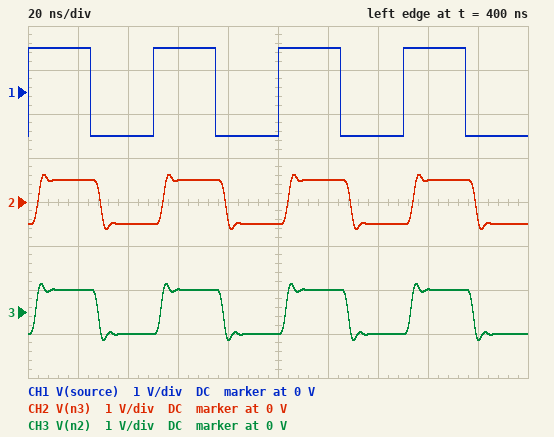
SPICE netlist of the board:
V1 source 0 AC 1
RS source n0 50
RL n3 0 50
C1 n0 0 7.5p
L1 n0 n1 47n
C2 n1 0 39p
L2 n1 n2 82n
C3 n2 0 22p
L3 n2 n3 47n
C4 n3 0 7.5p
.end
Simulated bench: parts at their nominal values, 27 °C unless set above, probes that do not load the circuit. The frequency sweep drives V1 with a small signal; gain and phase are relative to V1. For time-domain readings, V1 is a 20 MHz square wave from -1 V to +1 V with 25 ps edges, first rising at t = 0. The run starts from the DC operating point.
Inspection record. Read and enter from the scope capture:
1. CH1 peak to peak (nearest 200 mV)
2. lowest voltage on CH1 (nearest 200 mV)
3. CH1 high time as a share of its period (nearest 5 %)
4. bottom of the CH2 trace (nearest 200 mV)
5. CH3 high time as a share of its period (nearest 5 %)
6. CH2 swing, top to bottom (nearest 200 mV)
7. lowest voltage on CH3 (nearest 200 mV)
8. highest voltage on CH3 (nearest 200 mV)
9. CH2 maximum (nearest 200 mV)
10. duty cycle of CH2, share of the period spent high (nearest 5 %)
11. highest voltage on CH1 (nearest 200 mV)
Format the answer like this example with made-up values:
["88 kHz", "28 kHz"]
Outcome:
["2.0 V", "-1.0 V", "50 %", "-600 mV", "50 %", "1.2 V", "-600 mV", "600 mV", "600 mV", "50 %", "1.0 V"]
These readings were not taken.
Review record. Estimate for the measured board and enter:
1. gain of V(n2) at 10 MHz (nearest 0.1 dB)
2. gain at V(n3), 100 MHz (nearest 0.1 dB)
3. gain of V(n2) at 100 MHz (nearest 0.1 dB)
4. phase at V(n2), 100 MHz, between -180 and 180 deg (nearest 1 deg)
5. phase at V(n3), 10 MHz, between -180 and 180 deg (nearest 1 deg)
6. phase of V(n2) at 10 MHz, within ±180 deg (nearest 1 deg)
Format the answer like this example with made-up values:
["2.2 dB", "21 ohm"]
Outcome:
["-6.0 dB", "-6.3 dB", "-6.0 dB", "-103 deg", "-13 deg", "-10 deg"]
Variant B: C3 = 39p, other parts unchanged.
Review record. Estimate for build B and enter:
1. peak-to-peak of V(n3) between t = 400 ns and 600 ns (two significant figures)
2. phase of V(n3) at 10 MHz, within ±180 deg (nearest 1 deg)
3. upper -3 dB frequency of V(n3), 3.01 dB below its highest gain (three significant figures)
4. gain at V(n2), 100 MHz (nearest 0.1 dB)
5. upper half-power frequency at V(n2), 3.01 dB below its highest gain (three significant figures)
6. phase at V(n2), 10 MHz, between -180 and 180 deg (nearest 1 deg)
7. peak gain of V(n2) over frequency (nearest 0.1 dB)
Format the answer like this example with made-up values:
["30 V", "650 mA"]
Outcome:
["1.3 V", "-15 deg", "161 MHz", "-5.7 dB", "166 MHz", "-11 deg", "-5.5 dB"]
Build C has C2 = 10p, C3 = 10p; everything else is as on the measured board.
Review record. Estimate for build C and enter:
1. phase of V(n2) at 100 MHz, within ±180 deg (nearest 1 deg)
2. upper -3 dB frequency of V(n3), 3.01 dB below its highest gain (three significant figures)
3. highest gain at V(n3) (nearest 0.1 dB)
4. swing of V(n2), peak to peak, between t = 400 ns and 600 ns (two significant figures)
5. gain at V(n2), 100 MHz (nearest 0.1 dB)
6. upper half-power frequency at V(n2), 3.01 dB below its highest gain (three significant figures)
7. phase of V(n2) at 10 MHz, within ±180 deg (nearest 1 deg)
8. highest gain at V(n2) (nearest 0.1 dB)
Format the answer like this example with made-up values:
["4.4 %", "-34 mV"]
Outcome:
["-57 deg", "369 MHz", "-6.0 dB", "1.5 V", "-6.7 dB", "374 MHz", "-6 deg", "0.4 dB"]
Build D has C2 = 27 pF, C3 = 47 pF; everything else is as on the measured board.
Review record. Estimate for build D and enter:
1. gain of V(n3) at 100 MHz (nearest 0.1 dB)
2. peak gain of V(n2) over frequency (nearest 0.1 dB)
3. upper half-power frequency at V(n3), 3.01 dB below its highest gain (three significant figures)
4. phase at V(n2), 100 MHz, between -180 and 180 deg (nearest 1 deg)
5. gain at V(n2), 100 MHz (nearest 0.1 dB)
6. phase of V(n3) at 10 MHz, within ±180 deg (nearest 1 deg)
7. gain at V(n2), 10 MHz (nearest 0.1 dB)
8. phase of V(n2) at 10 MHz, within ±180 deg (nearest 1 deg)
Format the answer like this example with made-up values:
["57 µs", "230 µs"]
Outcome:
["-6.5 dB", "-6.0 dB", "161 MHz", "-115 deg", "-6.1 dB", "-14 deg", "-6.0 dB", "-11 deg"]
